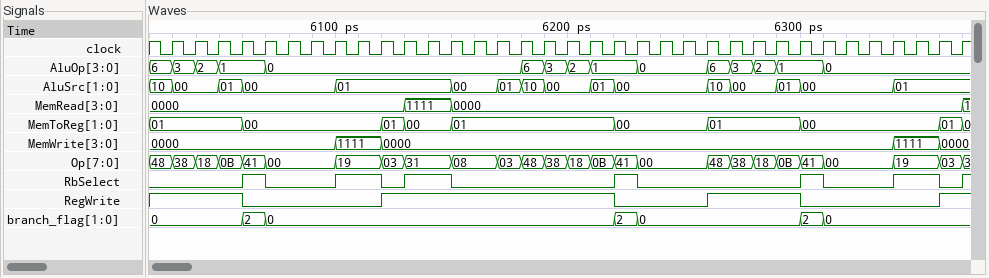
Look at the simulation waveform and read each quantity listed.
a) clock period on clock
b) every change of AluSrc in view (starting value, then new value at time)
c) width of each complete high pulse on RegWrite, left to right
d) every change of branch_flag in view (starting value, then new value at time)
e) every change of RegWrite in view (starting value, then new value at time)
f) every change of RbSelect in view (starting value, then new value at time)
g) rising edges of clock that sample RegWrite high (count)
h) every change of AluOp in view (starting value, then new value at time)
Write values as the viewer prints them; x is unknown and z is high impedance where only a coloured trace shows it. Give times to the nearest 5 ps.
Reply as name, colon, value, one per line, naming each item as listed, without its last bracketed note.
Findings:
clock period on clock: 10 ps
every change of AluSrc in view: 10, 00 at 6030 ps, 01 at 6050 ps, 00 at 6060 ps, 01 at 6100 ps, 00 at 6150 ps, 01 at 6170 ps, 10 at 6180 ps, 00 at 6190 ps, 01 at 6210 ps, 00 at 6220 ps, 10 at 6260 ps, 00 at 6270 ps, 01 at 6290 ps, 00 at 6300 ps, 01 at 6340 ps
width of each complete high pulse on RegWrite, left to right: 100 ps, 40 ps
every change of branch_flag in view: 0, 2 at 6060 ps, 0 at 6070 ps, 2 at 6220 ps, 0 at 6230 ps, 2 at 6300 ps, 0 at 6310 ps
every change of RegWrite in view: 1, 0 at 6060 ps, 1 at 6120 ps, 0 at 6220 ps, 1 at 6260 ps, 0 at 6300 ps, 1 at 6360 ps
every change of RbSelect in view: 0, 1 at 6060 ps, 0 at 6070 ps, 1 at 6100 ps, 0 at 6120 ps, 1 at 6130 ps, 0 at 6150 ps, 1 at 6220 ps, 0 at 6230 ps, 1 at 6300 ps, 0 at 6310 ps, 1 at 6340 ps, 0 at 6360 ps, 1 at 6370 ps
rising edges of clock that sample RegWrite high: 19
every change of AluOp in view: 6, 3 at 6030 ps, 2 at 6040 ps, 1 at 6050 ps, 0 at 6070 ps, 6 at 6180 ps, 3 at 6190 ps, 2 at 6200 ps, 1 at 6210 ps, 0 at 6230 ps, 6 at 6260 ps, 3 at 6270 ps, 2 at 6280 ps, 1 at 6290 ps, 0 at 6310 ps
